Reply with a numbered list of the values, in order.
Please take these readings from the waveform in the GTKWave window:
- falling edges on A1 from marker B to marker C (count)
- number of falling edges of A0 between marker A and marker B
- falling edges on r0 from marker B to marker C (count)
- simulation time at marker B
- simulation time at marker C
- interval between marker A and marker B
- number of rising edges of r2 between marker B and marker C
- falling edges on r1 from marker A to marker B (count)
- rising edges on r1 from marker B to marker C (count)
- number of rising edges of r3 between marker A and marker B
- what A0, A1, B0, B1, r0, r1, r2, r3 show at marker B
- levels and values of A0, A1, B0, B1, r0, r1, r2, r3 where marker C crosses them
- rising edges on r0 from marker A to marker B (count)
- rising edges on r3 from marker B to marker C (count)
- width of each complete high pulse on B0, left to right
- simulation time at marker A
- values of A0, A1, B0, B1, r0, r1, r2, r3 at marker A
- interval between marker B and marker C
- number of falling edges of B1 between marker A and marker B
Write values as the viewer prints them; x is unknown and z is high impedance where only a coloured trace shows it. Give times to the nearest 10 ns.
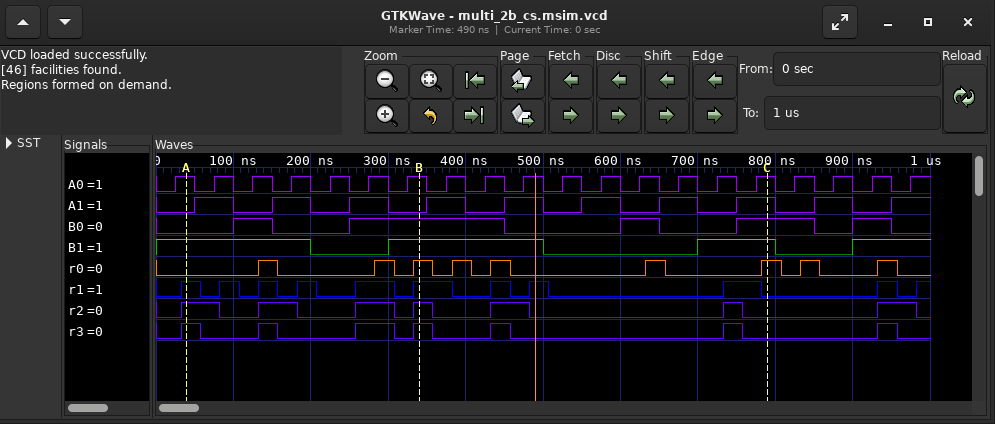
1. 4
2. 6
3. 4
4. 340 ns
5. 790 ns
6. 300 ns
7. 2
8. 5
9. 3
10. 3
11. A0=1, A1=0, B0=1, B1=1, r0=1, r1=1, r2=1, r3=1
12. A0=1, A1=1, B0=1, B1=1, r0=1, r1=0, r2=0, r3=0
13. 3
14. 2
15. 50 ns, 200 ns, 50 ns, 100 ns, 50 ns
16. 40 ns
17. A0=1, A1=0, B0=0, B1=1, r0=0, r1=1, r2=1, r3=1
18. 450 ns
19. 1
